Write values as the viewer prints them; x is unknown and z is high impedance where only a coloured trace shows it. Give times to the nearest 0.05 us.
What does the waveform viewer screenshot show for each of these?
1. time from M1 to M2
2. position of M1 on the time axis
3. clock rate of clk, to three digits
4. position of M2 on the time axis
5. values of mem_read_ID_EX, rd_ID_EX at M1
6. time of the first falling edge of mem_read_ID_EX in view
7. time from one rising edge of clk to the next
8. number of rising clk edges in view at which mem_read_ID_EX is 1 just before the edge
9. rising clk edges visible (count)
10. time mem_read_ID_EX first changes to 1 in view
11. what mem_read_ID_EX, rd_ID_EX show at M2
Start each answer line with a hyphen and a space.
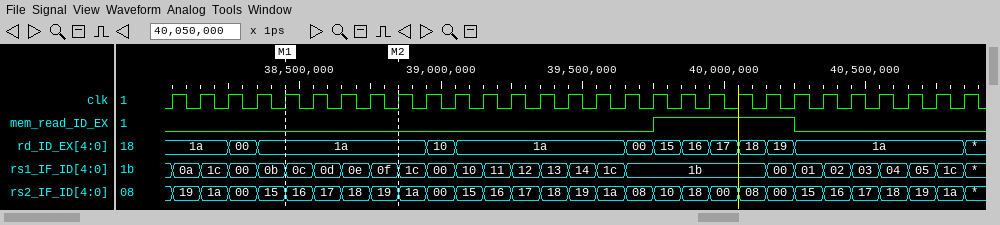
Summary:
- 0.4 us
- 38.45 us
- 10.0 MHz
- 38.85 us
- mem_read_ID_EX=0, rd_ID_EX=1a
- 40.25 us
- 0.1 us
- 5
- 29
- 39.75 us
- mem_read_ID_EX=0, rd_ID_EX=1a
